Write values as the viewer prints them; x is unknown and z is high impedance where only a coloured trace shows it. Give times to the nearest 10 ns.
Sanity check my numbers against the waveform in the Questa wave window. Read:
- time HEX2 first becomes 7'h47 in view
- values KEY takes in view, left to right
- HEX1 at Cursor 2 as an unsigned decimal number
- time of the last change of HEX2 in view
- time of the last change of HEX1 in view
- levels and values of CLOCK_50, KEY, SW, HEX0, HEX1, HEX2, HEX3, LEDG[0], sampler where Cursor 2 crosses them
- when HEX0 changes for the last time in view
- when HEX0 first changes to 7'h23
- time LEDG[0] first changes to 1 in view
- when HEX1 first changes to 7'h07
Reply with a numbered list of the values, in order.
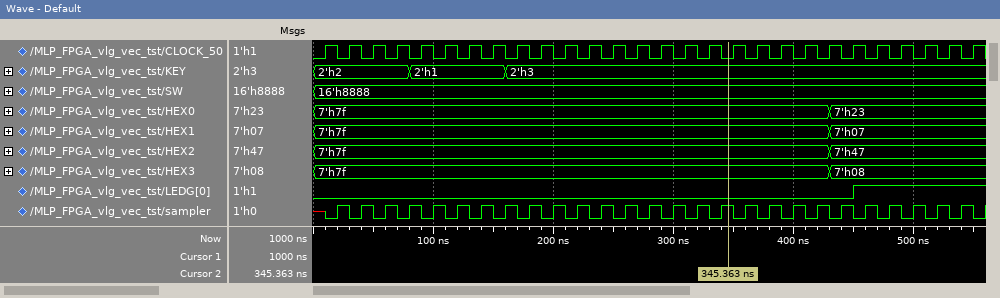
1. 430 ns
2. 2'h2, 2'h1, 2'h3
3. 127
4. 430 ns
5. 430 ns
6. CLOCK_50=0, KEY=2'h3, SW=16'h8888, HEX0=7'h7f, HEX1=7'h7f, HEX2=7'h7f, HEX3=7'h7f, LEDG[0]=0, sampler=1
7. 430 ns
8. 430 ns
9. 450 ns
10. 430 ns
